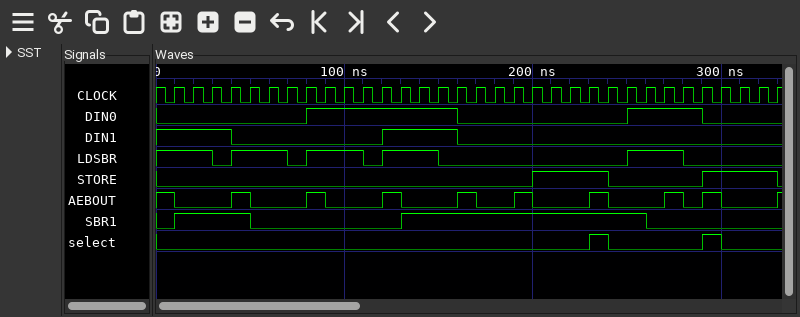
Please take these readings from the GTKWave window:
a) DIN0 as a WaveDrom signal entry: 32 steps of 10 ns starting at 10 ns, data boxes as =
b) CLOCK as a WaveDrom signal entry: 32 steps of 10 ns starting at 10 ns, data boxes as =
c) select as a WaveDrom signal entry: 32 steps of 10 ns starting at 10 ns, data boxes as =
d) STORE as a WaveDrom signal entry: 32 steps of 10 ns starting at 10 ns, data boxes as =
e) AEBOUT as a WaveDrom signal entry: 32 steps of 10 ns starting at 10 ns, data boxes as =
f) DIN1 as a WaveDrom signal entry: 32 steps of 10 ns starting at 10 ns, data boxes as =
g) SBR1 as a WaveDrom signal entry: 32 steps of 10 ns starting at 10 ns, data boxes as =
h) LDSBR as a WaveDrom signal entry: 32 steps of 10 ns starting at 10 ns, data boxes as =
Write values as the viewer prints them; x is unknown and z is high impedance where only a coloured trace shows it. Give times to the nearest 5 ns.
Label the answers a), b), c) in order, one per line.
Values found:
a) {name: 'DIN0', wave: '0......1.......0........1...0...'}
b) {name: 'CLOCK', wave: 'p...............................'}
c) {name: 'select', wave: '0.....................10....10..'}
d) {name: 'STORE', wave: '0..................1...0....1...'}
e) {name: 'AEBOUT', wave: '0..10..10..10..10.10..10..1010..'}
f) {name: 'DIN1', wave: '1..0.......1...0................'}
g) {name: 'SBR1', wave: '1...0.......1............0......'}
h) {name: 'LDSBR', wave: '1.01..01..01..0.........1..0....'}
